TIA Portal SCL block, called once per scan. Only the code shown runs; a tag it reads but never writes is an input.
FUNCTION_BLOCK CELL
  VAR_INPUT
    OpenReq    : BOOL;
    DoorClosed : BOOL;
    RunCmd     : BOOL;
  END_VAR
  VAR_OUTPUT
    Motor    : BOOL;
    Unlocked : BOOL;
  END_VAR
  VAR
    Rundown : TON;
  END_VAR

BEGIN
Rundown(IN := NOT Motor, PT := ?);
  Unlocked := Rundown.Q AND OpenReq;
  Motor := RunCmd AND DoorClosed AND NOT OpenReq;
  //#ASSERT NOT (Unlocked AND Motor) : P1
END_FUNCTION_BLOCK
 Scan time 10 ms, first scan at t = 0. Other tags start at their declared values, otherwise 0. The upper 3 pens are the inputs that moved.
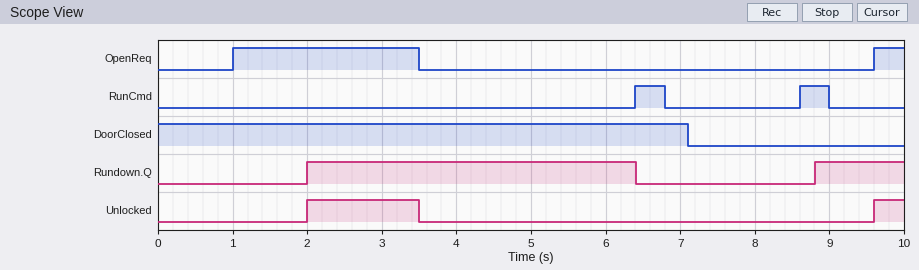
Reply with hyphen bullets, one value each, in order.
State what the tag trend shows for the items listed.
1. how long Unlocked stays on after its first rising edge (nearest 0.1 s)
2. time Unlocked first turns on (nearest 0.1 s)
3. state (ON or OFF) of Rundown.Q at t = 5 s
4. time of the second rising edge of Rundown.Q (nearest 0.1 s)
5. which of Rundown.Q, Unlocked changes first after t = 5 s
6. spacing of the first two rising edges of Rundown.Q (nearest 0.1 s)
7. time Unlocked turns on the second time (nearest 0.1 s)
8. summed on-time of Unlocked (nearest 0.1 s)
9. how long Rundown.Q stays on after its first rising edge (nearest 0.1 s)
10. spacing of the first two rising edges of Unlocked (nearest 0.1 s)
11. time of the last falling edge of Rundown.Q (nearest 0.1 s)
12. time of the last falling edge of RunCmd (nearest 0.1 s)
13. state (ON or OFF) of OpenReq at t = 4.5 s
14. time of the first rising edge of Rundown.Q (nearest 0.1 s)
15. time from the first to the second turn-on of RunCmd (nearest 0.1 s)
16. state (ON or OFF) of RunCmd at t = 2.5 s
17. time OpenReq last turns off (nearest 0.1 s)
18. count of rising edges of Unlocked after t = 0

- 1.5 s
- 2.0 s
- ON
- 8.8 s
- Rundown.Q
- 6.8 s
- 9.6 s
- 1.9 s
- 4.4 s
- 7.6 s
- 6.4 s
- 9.0 s
- OFF
- 2.0 s
- 2.2 s
- OFF
- 3.5 s
- 2
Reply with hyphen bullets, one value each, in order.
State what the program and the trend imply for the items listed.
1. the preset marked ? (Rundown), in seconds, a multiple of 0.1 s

- 2.0 s
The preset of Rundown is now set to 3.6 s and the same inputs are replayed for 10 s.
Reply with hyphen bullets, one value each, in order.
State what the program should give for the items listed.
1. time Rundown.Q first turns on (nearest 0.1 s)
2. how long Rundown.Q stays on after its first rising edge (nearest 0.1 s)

- 3.6 s
- 2.8 s
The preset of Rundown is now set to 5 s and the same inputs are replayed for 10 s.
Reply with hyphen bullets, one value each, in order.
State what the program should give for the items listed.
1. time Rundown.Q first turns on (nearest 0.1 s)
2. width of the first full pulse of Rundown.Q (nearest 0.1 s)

- 5.0 s
- 1.4 s
